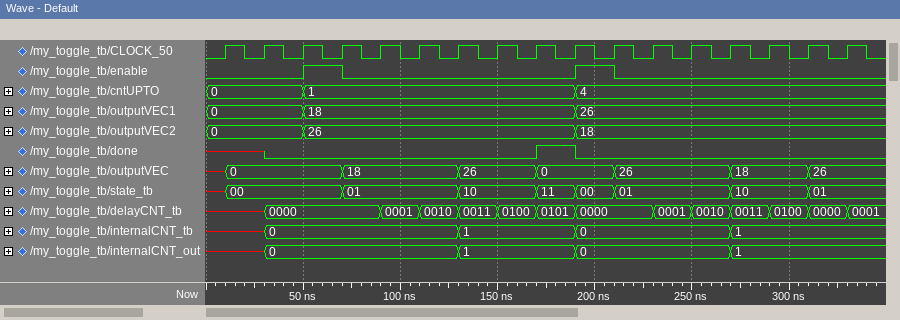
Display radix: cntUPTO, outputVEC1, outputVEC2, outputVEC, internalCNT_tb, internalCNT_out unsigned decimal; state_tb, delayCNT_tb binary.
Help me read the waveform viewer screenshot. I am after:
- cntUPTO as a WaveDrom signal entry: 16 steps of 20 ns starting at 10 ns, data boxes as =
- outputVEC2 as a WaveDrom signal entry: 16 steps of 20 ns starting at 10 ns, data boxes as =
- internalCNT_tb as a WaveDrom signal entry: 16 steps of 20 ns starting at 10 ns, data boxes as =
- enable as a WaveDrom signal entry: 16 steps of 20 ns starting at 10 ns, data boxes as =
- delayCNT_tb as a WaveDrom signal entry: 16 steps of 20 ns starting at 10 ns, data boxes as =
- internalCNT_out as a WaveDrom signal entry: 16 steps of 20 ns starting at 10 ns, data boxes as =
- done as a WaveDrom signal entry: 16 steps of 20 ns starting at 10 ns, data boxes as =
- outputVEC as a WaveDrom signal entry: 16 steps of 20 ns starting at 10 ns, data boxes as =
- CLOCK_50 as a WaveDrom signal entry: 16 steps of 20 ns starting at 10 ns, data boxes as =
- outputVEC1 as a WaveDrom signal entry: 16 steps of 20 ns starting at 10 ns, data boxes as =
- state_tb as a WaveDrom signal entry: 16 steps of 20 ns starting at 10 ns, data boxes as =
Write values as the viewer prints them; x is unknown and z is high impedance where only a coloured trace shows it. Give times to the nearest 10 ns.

{name: 'cntUPTO', wave: '=.=......=......', data: '0 1 4'}
{name: 'outputVEC2', wave: '=.=......=......', data: '0 26 18'}
{name: 'internalCNT_tb', wave: 'x=....=..=...=..', data: '0 1 0 1'}
{name: 'enable', wave: '0.10.....10.....'}
{name: 'delayCNT_tb', wave: 'x=..======.=====', data: '0000 0001 0010 0011 0100 0101 0000 0001 0010 0011 0100 0000'}
{name: 'internalCNT_out', wave: 'x=....=..=...=..', data: '0 1 0 1'}
{name: 'done', wave: 'x0......10......'}
{name: 'outputVEC', wave: '=..=..=.=.=..=.=', data: '0 18 26 0 26 18 26'}
{name: 'CLOCK_50', wave: 'p...............'}
{name: 'outputVEC1', wave: '=.=......=......', data: '0 18 26'}
{name: 'state_tb', wave: '=..=..=.===..=.=', data: '00 01 10 11 00 01 10 01'}
